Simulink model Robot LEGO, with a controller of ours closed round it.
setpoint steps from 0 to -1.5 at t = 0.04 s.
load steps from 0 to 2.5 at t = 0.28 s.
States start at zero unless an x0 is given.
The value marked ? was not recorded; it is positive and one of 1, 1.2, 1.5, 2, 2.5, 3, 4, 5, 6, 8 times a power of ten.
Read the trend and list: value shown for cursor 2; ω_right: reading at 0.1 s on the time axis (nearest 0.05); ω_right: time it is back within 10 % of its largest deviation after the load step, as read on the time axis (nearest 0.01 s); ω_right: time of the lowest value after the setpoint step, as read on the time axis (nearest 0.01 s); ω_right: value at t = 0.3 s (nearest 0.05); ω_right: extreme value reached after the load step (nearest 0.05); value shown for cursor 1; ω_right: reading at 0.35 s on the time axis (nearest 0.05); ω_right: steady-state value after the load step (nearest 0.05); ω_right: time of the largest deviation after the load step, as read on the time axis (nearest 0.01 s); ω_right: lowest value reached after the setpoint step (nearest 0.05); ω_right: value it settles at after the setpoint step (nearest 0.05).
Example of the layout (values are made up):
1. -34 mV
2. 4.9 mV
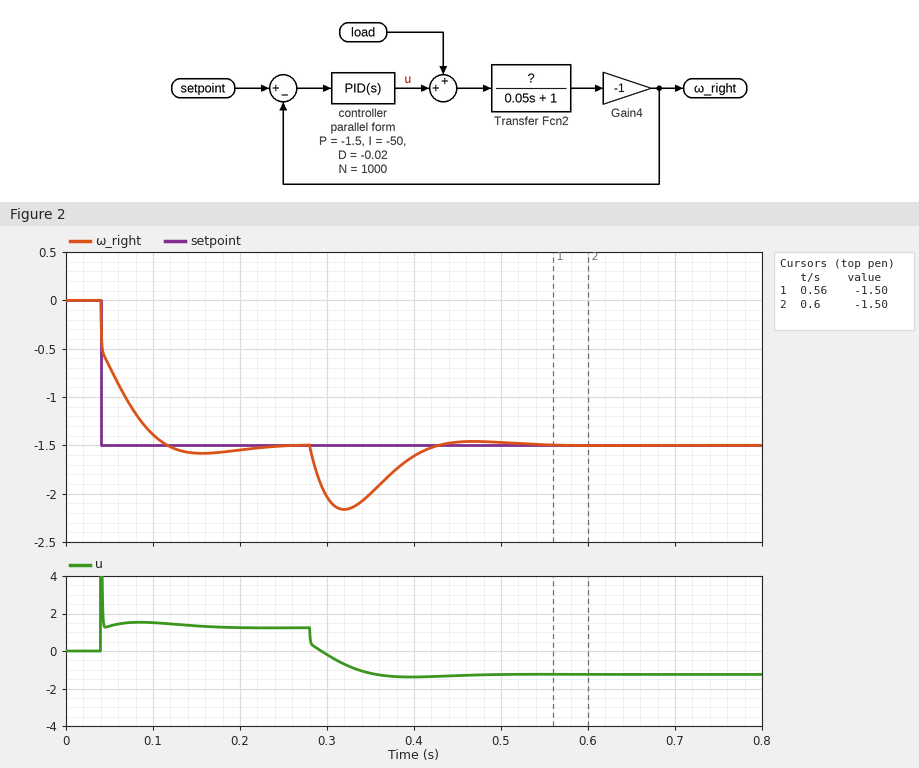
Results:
1. -1.50
2. -1.40
3. 0.41 s
4. 0.16 s
5. -2.05
6. -2.15
7. -1.50
8. -2.00
9. -1.50
10. 0.32 s
11. -1.60
12. -1.50
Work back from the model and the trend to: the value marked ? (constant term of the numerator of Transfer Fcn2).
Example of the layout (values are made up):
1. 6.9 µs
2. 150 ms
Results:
1. 1.2
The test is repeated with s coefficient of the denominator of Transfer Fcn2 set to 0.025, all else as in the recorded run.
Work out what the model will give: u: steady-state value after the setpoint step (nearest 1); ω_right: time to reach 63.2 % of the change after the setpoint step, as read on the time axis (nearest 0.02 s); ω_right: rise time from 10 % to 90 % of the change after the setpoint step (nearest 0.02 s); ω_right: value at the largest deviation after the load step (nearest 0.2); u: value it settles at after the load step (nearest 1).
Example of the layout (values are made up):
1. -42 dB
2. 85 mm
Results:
1. 1
2. 0.06 s
3. 0.06 s
4. -2.2
5. -1
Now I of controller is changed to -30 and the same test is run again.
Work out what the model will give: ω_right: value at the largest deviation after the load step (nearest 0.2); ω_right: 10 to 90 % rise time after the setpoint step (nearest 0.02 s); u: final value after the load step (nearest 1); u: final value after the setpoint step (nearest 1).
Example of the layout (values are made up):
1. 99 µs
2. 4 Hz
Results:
1. -2.2
2. 0.08 s
3. -1
4. 1
